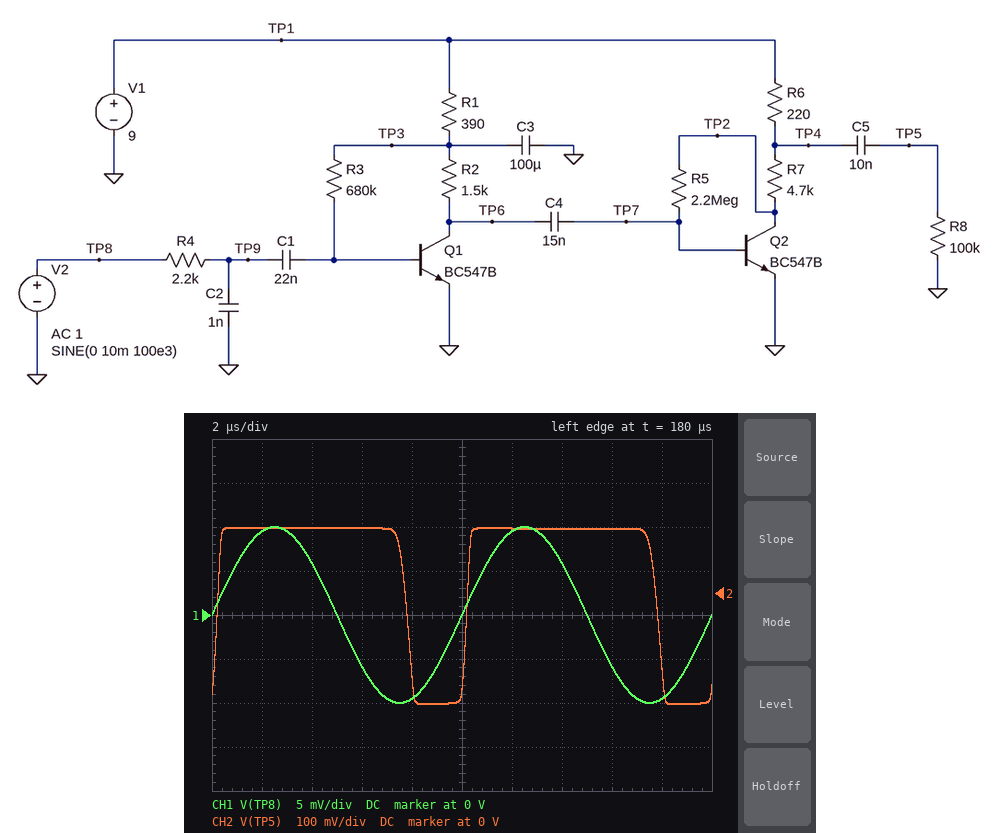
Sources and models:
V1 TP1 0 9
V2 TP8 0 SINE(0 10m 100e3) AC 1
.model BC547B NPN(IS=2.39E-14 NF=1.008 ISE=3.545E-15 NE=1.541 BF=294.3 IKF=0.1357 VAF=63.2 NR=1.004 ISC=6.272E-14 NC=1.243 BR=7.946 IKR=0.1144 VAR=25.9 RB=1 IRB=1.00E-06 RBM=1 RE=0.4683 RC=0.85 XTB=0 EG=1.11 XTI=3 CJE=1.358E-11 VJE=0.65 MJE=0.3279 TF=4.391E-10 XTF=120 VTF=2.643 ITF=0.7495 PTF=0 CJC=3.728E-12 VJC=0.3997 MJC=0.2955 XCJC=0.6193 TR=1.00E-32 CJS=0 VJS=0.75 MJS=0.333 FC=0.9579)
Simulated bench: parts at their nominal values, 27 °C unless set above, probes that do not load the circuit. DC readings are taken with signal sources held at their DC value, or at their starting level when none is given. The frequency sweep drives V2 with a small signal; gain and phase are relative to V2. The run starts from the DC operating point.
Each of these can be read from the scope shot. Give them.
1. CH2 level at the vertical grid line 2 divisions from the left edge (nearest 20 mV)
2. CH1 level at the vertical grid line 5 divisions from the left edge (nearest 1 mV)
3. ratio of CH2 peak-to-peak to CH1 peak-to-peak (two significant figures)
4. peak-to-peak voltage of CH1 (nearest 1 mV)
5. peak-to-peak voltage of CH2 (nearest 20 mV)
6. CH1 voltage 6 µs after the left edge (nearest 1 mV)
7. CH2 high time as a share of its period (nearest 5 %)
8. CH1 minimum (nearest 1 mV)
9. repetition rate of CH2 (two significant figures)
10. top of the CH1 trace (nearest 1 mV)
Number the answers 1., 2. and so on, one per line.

1. 140 mV
2. 0 V
3. 20
4. 20 mV
5. 400 mV
6. -6 mV
7. 75 %
8. -10 mV
9. 100 kHz
10. 10 mV
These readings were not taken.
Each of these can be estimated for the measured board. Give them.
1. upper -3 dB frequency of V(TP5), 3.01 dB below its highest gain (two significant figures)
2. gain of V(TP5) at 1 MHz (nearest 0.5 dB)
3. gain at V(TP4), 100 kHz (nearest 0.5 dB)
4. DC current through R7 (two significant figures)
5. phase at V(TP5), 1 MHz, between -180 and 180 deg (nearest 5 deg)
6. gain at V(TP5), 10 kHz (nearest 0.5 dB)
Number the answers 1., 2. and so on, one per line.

1. 96 kHz
2. 25.5 dB
3. 48.0 dB
4. 690 µA
5. -140 deg
6. 51.0 dB
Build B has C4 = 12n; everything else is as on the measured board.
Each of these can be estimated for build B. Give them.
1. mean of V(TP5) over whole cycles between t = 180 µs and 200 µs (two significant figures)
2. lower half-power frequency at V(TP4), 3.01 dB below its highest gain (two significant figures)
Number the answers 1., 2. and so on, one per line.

1. 57 mV
2. 2.3 kHz
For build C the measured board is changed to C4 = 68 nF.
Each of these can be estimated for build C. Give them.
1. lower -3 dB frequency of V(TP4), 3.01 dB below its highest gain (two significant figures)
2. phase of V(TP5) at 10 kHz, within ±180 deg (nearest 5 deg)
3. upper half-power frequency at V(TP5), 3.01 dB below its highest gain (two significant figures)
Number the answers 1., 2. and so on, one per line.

1. 1.5 kHz
2. 5 deg
3. 95 kHz
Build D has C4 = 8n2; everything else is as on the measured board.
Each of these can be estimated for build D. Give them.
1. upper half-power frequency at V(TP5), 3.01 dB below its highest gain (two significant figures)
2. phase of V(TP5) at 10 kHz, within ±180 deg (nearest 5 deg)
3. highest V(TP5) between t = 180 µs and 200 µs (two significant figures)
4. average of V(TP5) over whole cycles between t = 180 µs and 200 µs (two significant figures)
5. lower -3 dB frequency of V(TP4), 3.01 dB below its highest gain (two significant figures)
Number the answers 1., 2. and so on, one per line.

1. 97 kHz
2. 15 deg
3. 140 mV
4. 64 mV
5. 2.8 kHz
